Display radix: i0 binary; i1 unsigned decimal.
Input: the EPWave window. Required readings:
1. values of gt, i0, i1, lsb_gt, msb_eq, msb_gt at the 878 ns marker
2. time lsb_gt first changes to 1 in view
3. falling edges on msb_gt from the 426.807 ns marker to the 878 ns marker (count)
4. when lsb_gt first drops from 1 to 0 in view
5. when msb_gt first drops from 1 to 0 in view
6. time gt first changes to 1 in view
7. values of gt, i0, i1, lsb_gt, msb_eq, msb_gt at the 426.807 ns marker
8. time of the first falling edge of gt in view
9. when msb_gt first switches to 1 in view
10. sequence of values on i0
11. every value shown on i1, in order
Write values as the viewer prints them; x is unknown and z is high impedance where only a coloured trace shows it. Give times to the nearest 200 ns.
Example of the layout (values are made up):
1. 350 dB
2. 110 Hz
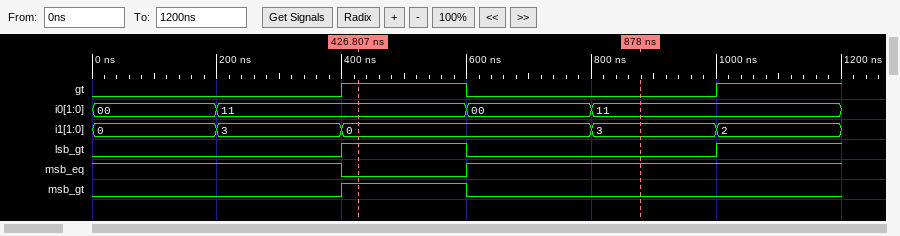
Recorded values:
1. gt=0, i0=11, i1=3, lsb_gt=0, msb_eq=1, msb_gt=0
2. 400 ns
3. 1
4. 600 ns
5. 600 ns
6. 400 ns
7. gt=1, i0=11, i1=0, lsb_gt=1, msb_eq=0, msb_gt=1
8. 600 ns
9. 400 ns
10. 00, 11, 00, 11
11. 0, 3, 0, 3, 2
